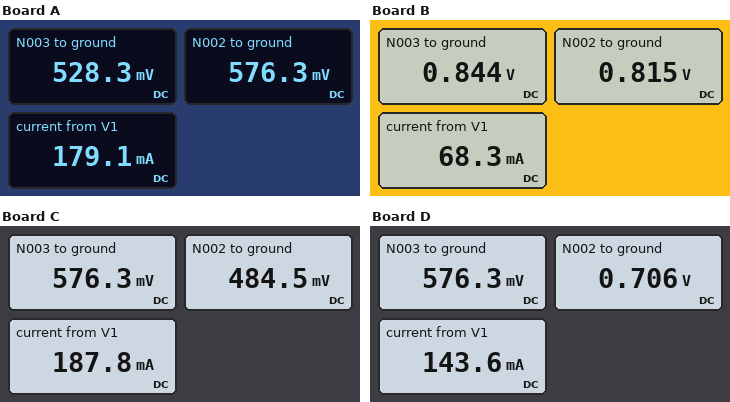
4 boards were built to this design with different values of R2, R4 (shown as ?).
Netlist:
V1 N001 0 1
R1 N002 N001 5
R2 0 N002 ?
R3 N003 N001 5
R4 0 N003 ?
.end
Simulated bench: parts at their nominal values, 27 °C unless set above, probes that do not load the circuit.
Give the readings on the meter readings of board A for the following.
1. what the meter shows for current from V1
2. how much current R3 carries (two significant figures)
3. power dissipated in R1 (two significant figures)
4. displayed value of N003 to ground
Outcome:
179.1 mA
94 mA
36 mW
528.3 mV
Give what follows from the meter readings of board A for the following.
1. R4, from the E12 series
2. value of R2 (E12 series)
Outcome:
5.6 Ω
6.8 Ω
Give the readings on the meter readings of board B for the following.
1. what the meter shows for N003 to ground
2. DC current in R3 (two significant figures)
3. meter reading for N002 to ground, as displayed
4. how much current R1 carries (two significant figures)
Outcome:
0.844 V
31 mA
0.815 V
37 mA
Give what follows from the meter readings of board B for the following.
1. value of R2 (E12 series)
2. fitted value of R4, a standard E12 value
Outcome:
22 Ω
27 Ω
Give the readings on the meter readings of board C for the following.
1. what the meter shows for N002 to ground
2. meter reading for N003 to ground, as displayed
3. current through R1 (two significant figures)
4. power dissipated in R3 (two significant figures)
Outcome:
484.5 mV
576.3 mV
100 mA
36 mW
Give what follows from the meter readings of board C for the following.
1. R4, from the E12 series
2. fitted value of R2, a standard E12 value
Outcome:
6.8 Ω
4.7 Ω
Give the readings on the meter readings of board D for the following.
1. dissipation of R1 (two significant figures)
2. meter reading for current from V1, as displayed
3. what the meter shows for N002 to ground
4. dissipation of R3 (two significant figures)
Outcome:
17 mW
143.6 mA
0.706 V
36 mW
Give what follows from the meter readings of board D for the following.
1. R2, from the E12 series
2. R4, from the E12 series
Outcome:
12 Ω
6.8 Ω
